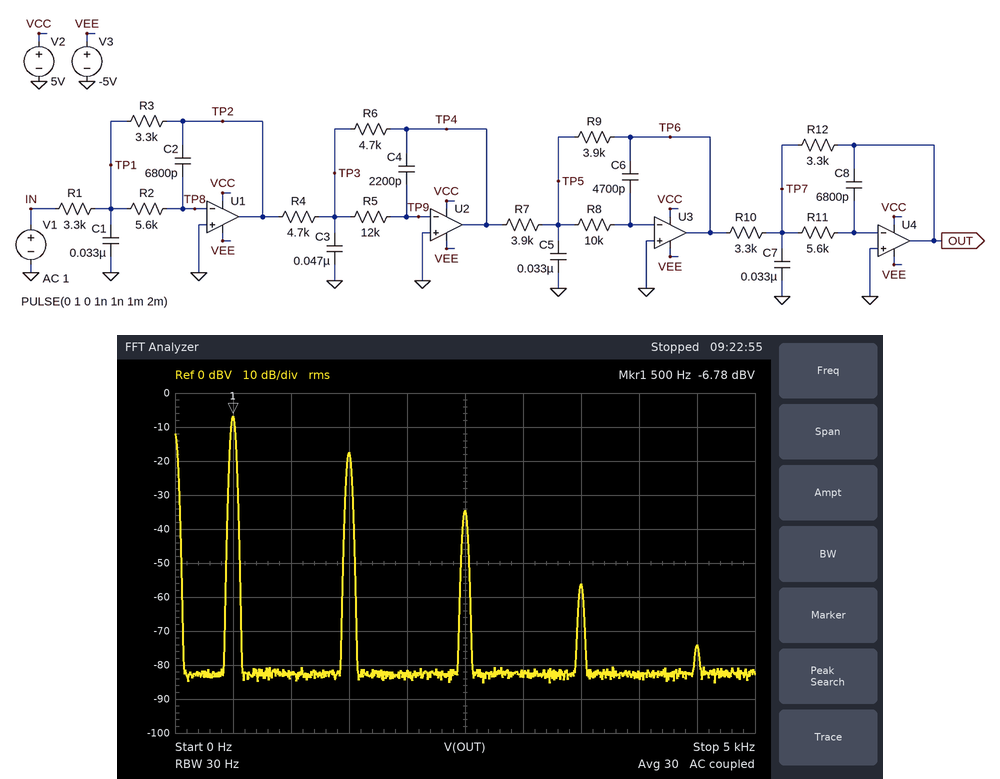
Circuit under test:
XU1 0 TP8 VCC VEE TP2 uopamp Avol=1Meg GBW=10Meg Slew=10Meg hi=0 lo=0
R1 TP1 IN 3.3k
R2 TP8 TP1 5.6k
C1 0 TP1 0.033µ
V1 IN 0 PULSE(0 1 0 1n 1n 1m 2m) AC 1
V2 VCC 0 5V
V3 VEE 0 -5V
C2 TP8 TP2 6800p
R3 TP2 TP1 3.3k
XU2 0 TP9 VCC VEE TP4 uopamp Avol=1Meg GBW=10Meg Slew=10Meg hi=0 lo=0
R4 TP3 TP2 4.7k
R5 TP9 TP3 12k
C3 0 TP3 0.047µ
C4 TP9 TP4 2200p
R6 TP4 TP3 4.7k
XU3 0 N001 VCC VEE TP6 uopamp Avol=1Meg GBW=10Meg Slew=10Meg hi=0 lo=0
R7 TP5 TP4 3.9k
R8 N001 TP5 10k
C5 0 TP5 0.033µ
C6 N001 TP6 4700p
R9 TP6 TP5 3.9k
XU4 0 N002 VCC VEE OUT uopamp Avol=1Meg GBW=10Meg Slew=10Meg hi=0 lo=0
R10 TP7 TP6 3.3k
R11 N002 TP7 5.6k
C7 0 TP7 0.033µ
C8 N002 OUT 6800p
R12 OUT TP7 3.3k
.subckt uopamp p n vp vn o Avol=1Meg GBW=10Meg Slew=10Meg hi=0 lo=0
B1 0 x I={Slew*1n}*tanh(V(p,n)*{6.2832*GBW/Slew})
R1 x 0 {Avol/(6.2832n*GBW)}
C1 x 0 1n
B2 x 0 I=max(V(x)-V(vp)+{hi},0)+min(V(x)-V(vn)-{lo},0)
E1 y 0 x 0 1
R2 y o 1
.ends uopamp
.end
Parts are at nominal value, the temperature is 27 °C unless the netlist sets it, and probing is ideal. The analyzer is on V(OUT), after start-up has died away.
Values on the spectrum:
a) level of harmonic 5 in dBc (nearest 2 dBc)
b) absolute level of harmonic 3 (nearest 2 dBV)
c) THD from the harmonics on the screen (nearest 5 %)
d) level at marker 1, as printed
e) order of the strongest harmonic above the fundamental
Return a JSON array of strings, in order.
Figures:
["-28 dBc", "-18 dBV", "30 %", "-6.78 dBV", "3"]
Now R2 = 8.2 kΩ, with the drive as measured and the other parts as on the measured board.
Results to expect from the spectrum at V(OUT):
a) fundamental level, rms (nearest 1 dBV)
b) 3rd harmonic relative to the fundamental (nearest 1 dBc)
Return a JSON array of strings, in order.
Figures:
["-7 dBV", "-12 dBc"]
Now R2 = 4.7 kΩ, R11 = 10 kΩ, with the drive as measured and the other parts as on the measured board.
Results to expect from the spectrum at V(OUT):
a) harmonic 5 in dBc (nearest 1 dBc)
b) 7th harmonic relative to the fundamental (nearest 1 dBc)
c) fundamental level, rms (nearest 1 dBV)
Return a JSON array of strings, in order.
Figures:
["-31 dBc", "-53 dBc", "-7 dBV"]
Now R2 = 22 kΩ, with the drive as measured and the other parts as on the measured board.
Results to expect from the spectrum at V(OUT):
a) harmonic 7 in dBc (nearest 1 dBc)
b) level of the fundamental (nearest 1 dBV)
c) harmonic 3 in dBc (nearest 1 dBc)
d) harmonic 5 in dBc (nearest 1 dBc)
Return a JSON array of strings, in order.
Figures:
["-59 dBc", "-9 dBV", "-17 dBc", "-37 dBc"]
